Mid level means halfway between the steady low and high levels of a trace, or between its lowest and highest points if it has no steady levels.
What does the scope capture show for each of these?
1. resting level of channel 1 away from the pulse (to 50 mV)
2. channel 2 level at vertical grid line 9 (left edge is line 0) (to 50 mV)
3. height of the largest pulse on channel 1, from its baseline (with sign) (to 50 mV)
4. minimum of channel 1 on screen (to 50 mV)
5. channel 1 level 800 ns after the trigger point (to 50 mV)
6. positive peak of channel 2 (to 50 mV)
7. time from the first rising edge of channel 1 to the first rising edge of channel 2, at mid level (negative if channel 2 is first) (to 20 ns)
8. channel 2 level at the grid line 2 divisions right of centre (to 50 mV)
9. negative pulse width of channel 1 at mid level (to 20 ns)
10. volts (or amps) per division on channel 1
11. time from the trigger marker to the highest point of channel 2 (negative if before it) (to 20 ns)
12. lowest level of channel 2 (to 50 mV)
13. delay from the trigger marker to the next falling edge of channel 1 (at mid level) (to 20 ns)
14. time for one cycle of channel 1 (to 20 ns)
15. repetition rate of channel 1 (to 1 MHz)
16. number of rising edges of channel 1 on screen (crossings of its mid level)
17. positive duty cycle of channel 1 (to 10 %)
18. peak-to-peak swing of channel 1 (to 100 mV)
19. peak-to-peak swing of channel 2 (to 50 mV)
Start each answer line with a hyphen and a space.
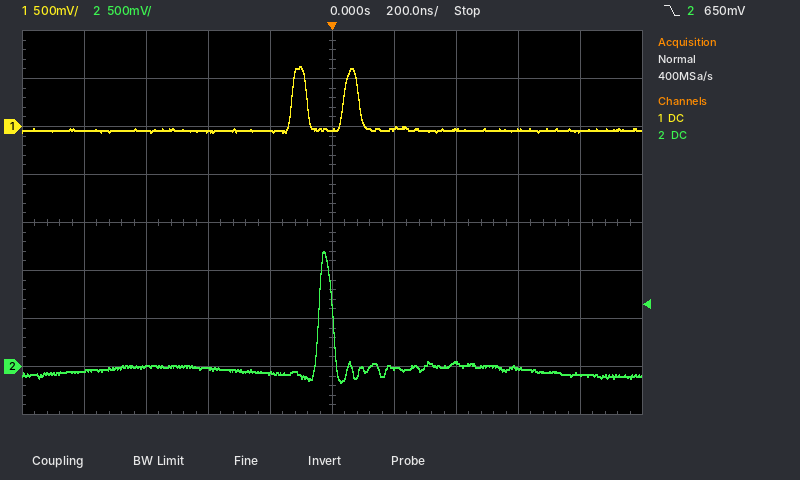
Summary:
- -50 mV
- -100 mV
- +650 mV
- -50 mV
- -50 mV
- 1.20 V
- +80 ns
- 50 mV
- 120 ns
- 500 mV
- -20 ns
- -150 mV
- 80 ns
- 160 ns
- 6 MHz
- 2
- 30 %
- 700 mV
- 1.35 V
